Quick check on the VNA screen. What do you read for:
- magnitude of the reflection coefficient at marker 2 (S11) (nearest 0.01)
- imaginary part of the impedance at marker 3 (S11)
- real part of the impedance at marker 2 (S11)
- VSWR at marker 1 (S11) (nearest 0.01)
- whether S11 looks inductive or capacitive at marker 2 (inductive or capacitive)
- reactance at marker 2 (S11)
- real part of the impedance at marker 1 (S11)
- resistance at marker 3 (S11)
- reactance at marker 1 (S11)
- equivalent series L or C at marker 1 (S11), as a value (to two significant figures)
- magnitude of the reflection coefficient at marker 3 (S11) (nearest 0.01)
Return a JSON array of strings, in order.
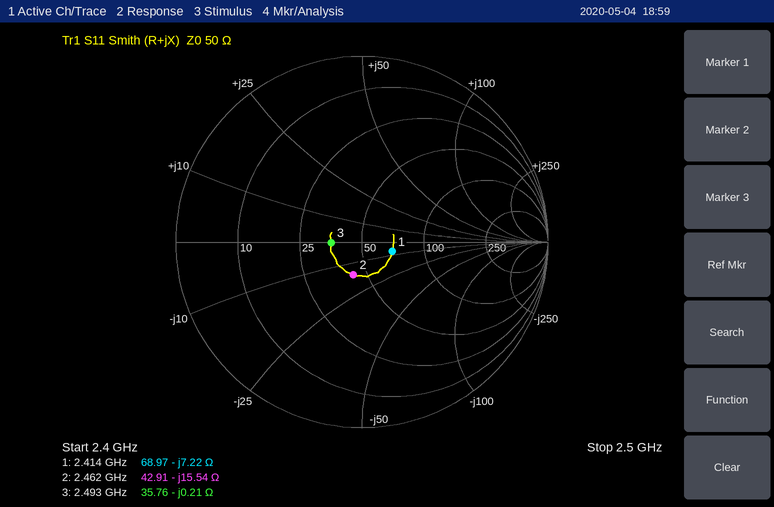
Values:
["0.18", "-0.21 Ω", "42.91 Ω", "1.41", "capacitive", "-15.54 Ω", "68.97 Ω", "35.76 Ω", "-7.22 Ω", "9.1 pF", "0.17"]
